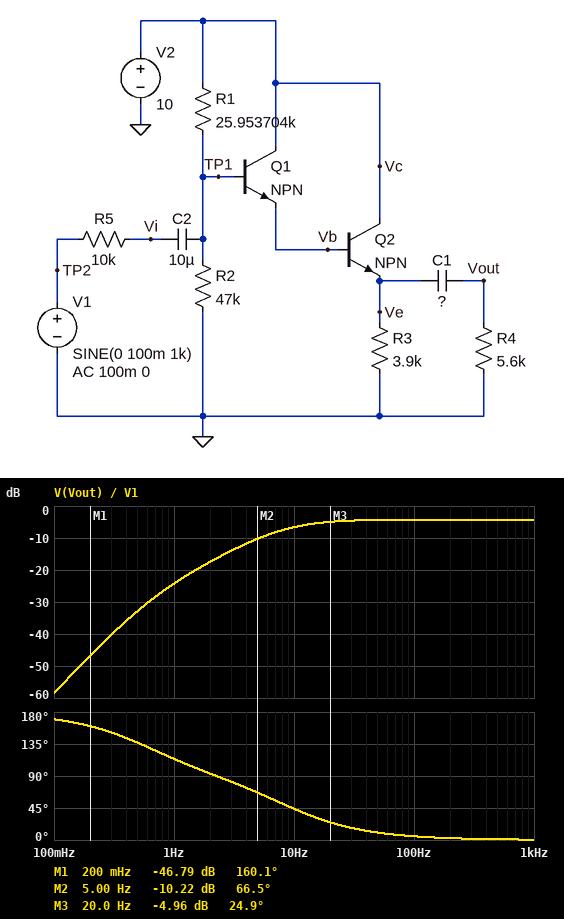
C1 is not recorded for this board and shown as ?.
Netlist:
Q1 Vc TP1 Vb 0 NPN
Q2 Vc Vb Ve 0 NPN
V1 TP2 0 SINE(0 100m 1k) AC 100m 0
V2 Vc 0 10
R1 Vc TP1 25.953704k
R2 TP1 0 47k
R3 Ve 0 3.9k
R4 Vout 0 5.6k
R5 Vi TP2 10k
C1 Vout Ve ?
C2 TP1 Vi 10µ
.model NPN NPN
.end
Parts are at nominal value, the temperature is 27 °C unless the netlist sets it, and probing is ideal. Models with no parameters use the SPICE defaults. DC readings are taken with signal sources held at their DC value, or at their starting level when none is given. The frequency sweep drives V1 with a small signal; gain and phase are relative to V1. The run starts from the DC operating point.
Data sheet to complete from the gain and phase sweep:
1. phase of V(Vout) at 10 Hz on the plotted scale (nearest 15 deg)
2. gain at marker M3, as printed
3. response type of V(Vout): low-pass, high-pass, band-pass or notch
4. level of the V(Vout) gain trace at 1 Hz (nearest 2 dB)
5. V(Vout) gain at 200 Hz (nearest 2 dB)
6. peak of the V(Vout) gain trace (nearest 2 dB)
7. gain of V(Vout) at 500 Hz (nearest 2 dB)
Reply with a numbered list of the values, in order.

1. 45 deg
2. -4.96 dB
3. high-pass
4. -24 dB
5. -4 dB
6. -4 dB
7. -4 dB
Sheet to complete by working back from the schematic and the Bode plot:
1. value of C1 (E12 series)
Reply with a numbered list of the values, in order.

1. 3.3 µF
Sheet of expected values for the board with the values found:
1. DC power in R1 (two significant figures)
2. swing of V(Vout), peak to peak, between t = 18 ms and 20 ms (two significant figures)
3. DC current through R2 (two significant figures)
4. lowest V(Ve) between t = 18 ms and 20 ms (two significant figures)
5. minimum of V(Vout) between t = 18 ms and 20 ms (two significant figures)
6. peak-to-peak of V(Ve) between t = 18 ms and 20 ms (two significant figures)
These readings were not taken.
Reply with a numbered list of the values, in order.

1. 490 µW
2. 120 mV
3. 140 µA
4. 4.9 V
5. -62 mV
6. 120 mV
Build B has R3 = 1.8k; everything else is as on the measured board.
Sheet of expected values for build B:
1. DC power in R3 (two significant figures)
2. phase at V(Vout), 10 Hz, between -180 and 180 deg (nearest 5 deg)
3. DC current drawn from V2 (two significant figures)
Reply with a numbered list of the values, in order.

1. 14 mW
2. 45 deg
3. 2.9 mA
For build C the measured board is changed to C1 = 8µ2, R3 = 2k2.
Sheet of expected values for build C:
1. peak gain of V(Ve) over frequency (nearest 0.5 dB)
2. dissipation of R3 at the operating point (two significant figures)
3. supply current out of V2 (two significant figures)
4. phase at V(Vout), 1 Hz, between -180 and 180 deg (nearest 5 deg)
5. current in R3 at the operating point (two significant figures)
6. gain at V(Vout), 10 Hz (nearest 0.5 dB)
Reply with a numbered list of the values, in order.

1. -4.0 dB
2. 11 mW
3. 2.4 mA
4. 105 deg
5. 2.3 mA
6. -4.5 dB
